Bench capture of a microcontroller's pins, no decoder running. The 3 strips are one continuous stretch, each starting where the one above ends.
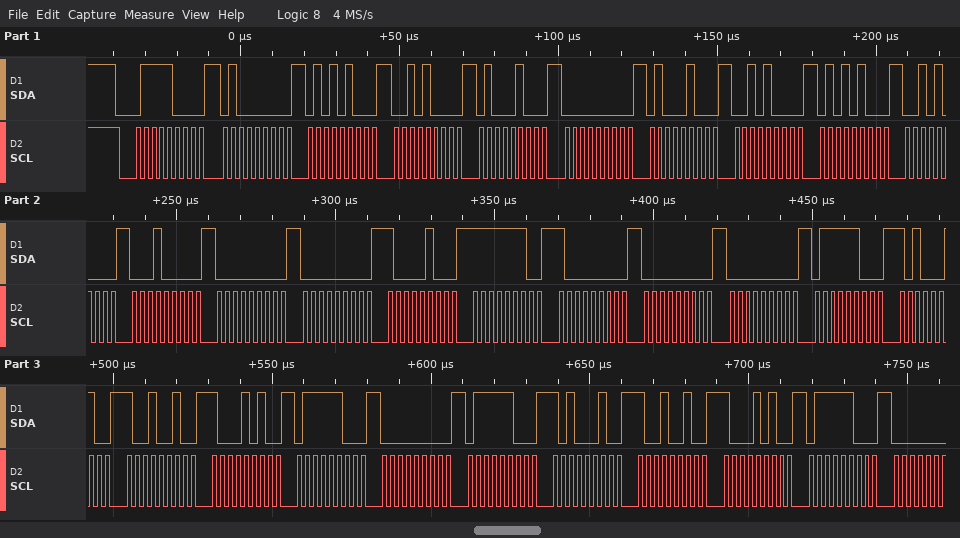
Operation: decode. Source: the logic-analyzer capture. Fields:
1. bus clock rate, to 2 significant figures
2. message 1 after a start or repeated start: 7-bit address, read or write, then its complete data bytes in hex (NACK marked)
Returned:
400 kHz
0x3C write: 40 54 28 44 00 44 28 54 28 10 00 00 84 FE 80 00 00 7C A2 92 8A 7C 00 7C A2 92 8A 7C
